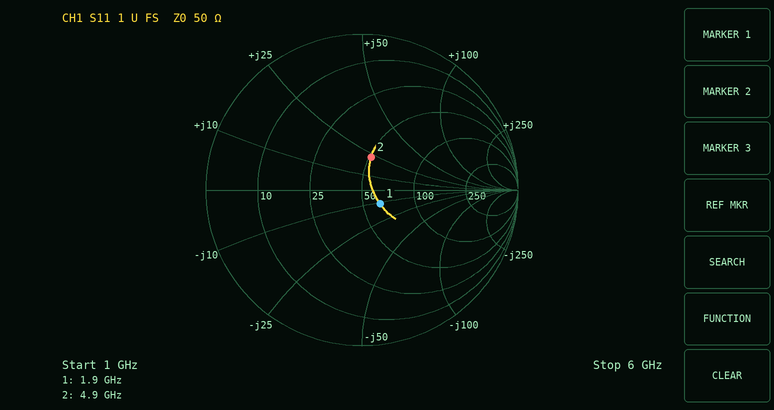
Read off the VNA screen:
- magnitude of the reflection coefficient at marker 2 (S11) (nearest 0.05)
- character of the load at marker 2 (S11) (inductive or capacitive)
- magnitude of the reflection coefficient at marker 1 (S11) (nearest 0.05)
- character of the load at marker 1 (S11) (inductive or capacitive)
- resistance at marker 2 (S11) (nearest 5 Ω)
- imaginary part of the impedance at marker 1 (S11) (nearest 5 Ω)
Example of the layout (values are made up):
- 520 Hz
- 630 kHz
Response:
- 0.20
- inductive
- 0.15
- capacitive
- 50 Ω
- -10 Ω
